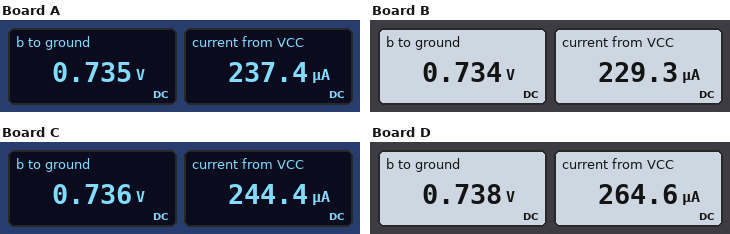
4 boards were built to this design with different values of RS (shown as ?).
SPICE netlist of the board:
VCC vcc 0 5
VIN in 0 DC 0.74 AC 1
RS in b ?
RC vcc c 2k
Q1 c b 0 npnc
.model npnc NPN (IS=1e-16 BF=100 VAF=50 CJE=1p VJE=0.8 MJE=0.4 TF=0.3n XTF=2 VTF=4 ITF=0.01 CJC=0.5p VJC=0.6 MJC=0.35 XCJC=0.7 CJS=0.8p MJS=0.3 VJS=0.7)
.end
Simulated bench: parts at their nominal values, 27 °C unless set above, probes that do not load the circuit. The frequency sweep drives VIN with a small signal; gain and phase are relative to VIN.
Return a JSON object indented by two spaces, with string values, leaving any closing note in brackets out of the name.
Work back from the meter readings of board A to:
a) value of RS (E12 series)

{
  "value of RS": "2.2 kΩ"
}
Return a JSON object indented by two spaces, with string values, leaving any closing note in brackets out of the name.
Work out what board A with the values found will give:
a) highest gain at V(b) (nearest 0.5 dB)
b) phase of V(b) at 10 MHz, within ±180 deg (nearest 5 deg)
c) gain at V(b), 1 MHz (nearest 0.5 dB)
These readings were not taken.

{
  "highest gain at V(b)": "-1.5 dB",
  "phase of V(b) at 10 MHz, within ±180 deg": "-45 deg",
  "gain at V(b), 1 MHz": "-1.5 dB"
}
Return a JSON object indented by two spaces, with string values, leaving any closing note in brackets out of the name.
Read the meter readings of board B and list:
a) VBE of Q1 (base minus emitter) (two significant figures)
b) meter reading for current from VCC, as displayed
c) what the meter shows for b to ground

{
  "VBE of Q1 (base minus emitter)": "730 mV",
  "meter reading for current from VCC, as displayed": "229.3 µA",
  "what the meter shows for b to ground": "0.734 V"
}
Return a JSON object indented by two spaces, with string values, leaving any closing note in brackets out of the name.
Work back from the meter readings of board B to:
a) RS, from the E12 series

{
  "RS, from the E12 series": "2.7 kΩ"
}
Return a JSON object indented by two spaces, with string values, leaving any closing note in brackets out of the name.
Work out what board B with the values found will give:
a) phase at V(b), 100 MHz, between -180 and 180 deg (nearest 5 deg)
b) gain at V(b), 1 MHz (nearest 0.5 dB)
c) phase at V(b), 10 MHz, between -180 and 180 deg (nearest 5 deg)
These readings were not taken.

{
  "phase at V(b), 100 MHz, between -180 and 180 deg": "-70 deg",
  "gain at V(b), 1 MHz": "-2.0 dB",
  "phase at V(b), 10 MHz, between -180 and 180 deg": "-50 deg"
}
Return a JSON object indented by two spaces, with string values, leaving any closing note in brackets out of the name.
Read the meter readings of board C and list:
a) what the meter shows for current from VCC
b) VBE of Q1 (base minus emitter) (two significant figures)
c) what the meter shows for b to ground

{
  "what the meter shows for current from VCC": "244.4 µA",
  "VBE of Q1 (base minus emitter)": "740 mV",
  "what the meter shows for b to ground": "0.736 V"
}
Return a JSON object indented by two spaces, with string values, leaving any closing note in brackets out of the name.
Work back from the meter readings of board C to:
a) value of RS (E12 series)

{
  "value of RS": "1.8 kΩ"
}
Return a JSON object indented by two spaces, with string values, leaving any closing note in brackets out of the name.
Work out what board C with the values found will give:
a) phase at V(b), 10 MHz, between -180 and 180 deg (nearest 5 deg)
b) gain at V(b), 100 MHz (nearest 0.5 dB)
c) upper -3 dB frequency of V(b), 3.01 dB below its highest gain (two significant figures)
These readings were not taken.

{
  "phase at V(b), 10 MHz, between -180 and 180 deg": "-40 deg",
  "gain at V(b), 100 MHz": "-19.5 dB",
  "upper -3 dB frequency of V(b), 3.01 dB below its highest gain": "10 MHz"
}
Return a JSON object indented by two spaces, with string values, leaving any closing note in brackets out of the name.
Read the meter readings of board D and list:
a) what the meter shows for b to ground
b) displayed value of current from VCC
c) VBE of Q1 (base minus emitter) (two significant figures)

{
  "what the meter shows for b to ground": "0.738 V",
  "displayed value of current from VCC": "264.6 µA",
  "VBE of Q1 (base minus emitter)": "740 mV"
}
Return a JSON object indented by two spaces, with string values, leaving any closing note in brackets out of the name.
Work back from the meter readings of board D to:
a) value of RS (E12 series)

{
  "value of RS": "820 Ω"
}
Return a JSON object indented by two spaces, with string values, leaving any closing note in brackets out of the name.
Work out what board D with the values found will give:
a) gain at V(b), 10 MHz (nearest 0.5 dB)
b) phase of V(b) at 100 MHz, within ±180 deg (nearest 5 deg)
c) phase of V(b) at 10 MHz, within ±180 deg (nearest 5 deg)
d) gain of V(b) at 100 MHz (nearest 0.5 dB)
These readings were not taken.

{
  "gain at V(b), 10 MHz": "-1.5 dB",
  "phase of V(b) at 100 MHz, within ±180 deg": "-60 deg",
  "phase of V(b) at 10 MHz, within ±180 deg": "-25 deg",
  "gain of V(b) at 100 MHz": "-13.5 dB"
}
